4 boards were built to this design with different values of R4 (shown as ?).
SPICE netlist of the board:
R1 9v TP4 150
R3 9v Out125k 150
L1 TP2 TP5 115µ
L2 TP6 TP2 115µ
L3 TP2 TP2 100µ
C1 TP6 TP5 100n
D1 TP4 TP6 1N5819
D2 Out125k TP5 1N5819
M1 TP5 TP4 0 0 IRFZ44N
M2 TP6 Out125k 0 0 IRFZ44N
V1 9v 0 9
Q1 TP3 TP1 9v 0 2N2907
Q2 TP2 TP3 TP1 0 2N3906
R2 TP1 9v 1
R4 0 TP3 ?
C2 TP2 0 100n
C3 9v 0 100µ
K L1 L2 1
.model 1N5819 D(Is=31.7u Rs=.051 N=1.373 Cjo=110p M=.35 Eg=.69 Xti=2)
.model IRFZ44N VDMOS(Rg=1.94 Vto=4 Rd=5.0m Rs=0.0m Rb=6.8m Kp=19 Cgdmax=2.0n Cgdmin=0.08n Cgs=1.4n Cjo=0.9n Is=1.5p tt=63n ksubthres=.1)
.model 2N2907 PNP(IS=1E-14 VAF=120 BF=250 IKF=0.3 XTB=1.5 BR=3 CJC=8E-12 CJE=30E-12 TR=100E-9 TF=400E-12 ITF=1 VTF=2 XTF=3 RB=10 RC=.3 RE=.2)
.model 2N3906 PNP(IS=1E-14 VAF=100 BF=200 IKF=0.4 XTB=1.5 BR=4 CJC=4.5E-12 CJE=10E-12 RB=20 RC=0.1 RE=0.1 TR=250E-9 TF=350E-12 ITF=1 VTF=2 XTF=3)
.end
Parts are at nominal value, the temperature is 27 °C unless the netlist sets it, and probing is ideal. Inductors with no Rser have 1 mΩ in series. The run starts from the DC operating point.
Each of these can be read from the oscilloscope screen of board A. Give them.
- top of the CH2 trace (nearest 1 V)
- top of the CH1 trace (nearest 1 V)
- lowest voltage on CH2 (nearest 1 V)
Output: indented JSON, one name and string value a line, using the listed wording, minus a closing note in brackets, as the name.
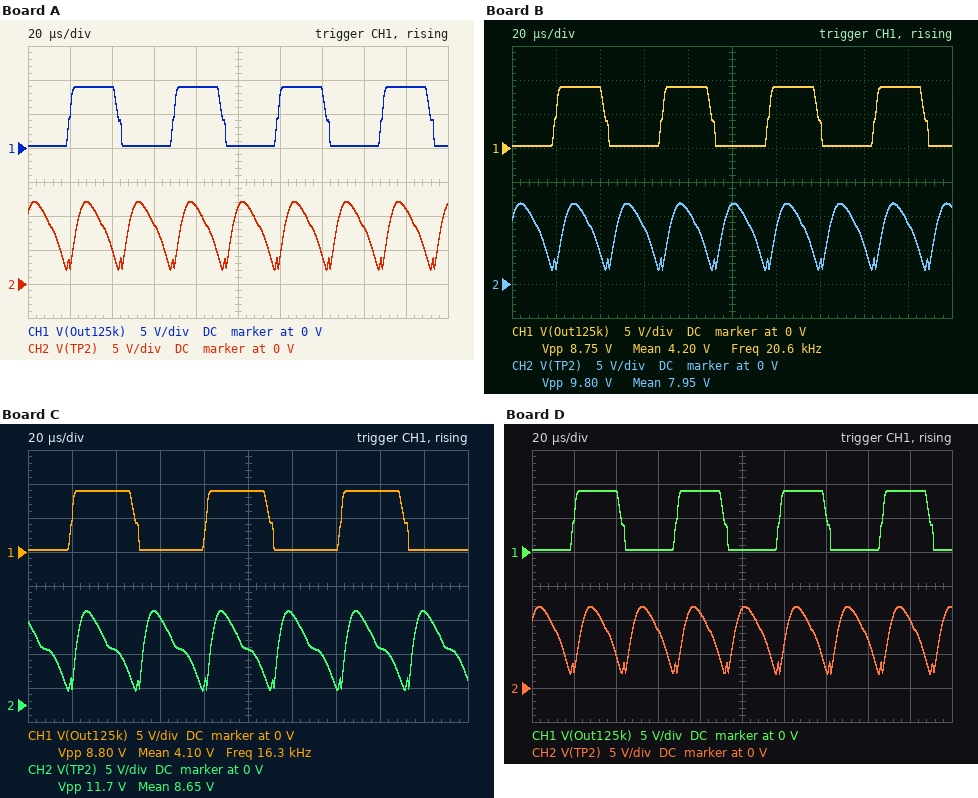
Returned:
{
  "top of the CH2 trace": "12 V",
  "top of the CH1 trace": "9 V",
  "lowest voltage on CH2": "2 V"
}
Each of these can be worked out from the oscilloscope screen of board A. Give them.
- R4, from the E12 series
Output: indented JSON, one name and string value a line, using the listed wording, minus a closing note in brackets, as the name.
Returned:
{
  "R4, from the E12 series": "4.7 kΩ"
}
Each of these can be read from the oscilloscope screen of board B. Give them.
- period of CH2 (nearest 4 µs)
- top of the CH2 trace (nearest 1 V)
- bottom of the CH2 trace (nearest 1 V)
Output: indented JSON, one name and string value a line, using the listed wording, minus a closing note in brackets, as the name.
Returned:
{
  "period of CH2": "24 µs",
  "top of the CH2 trace": "12 V",
  "bottom of the CH2 trace": "2 V"
}
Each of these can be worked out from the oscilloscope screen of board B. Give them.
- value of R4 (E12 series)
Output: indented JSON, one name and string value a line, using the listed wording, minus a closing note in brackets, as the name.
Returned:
{
  "value of R4": "6.8 kΩ"
}
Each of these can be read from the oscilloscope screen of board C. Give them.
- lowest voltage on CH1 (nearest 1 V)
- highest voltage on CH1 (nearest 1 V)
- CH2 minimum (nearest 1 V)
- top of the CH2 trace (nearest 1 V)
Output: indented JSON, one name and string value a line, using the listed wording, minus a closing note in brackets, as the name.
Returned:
{
  "lowest voltage on CH1": "0 V",
  "highest voltage on CH1": "9 V",
  "CH2 minimum": "2 V",
  "top of the CH2 trace": "14 V"
}
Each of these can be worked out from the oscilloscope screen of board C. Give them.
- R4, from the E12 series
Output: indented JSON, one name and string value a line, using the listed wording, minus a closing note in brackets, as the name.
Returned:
{
  "R4, from the E12 series": "1 kΩ"
}
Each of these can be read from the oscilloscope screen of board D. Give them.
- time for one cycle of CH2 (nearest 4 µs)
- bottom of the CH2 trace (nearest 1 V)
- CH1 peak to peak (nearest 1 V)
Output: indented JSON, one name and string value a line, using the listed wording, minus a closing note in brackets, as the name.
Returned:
{
  "time for one cycle of CH2": "24 µs",
  "bottom of the CH2 trace": "2 V",
  "CH1 peak to peak": "9 V"
}
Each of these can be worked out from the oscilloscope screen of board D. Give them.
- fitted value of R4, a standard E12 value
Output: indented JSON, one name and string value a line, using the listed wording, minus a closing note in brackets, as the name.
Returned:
{
  "fitted value of R4, a standard E12 value": "5.6 kΩ"
}
